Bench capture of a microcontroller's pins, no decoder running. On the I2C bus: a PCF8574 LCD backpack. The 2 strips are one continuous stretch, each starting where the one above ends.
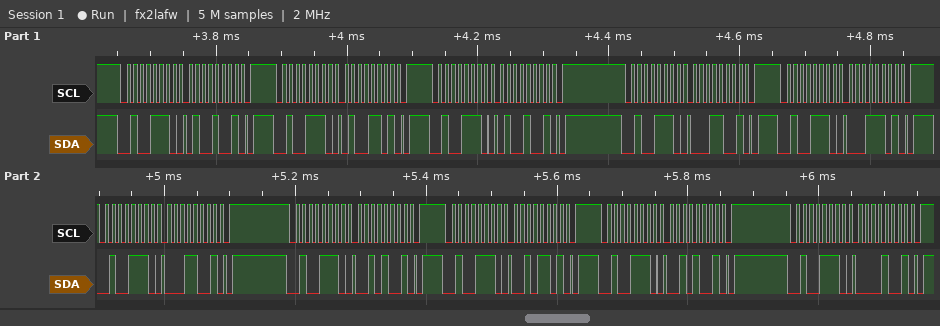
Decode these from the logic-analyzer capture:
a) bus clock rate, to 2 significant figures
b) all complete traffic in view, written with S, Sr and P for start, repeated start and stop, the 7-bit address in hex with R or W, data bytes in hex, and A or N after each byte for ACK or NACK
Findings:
100 kHz
S 27W A 49 A P S 27W A 4D A P S 27W A 49 A P S 27W A 19 A P S 27W A 1D A P S 27W A 19 A P S 27W A 29 A P S 27W A 2D A P S 27W A 29 A P S 27W A 09 A P
